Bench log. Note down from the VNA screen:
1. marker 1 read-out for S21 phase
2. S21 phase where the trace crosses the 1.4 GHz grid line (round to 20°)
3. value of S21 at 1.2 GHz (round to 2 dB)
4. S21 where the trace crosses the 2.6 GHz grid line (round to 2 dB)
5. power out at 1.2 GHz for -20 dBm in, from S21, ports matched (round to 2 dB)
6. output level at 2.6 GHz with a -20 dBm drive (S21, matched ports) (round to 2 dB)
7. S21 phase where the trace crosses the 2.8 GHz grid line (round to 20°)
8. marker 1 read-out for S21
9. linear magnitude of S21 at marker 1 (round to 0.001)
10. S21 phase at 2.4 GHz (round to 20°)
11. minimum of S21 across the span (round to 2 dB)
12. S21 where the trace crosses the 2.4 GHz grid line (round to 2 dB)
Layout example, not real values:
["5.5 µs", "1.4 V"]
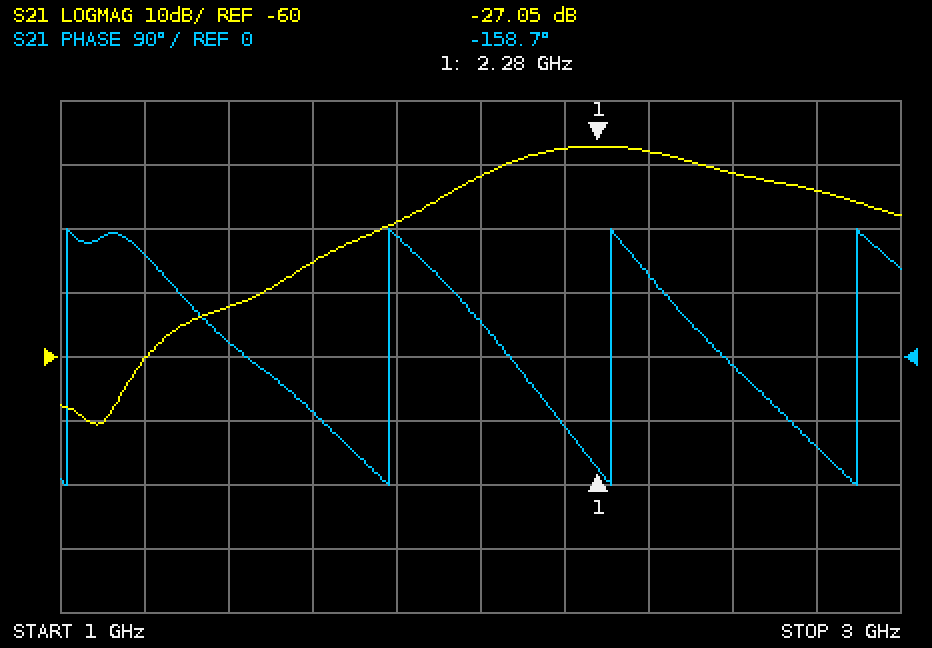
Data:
["-158.7°", "20°", "-60 dB", "-32 dB", "-80 dBm", "-52 dBm", "-120°", "-27.05 dB", "0.044", "120°", "-70 dB", "-28 dB"]
